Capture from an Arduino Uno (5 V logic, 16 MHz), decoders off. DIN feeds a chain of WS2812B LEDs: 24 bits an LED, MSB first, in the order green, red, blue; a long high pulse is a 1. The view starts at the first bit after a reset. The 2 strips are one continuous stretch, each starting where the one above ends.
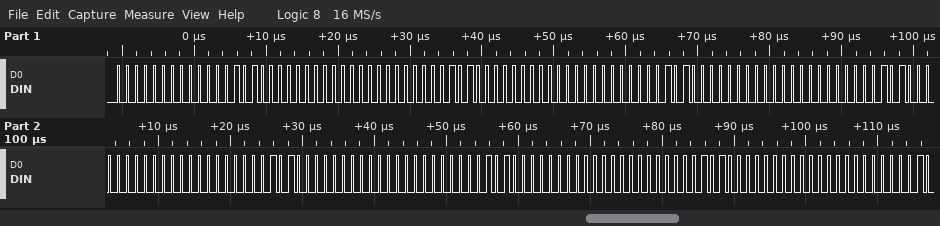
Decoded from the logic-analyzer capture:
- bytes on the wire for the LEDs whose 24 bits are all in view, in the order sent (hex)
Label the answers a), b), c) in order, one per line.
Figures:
a) 00 05 00 00 05 00 00 05 00 00 05 00 00 05 00 00 05 00 00 05 00
